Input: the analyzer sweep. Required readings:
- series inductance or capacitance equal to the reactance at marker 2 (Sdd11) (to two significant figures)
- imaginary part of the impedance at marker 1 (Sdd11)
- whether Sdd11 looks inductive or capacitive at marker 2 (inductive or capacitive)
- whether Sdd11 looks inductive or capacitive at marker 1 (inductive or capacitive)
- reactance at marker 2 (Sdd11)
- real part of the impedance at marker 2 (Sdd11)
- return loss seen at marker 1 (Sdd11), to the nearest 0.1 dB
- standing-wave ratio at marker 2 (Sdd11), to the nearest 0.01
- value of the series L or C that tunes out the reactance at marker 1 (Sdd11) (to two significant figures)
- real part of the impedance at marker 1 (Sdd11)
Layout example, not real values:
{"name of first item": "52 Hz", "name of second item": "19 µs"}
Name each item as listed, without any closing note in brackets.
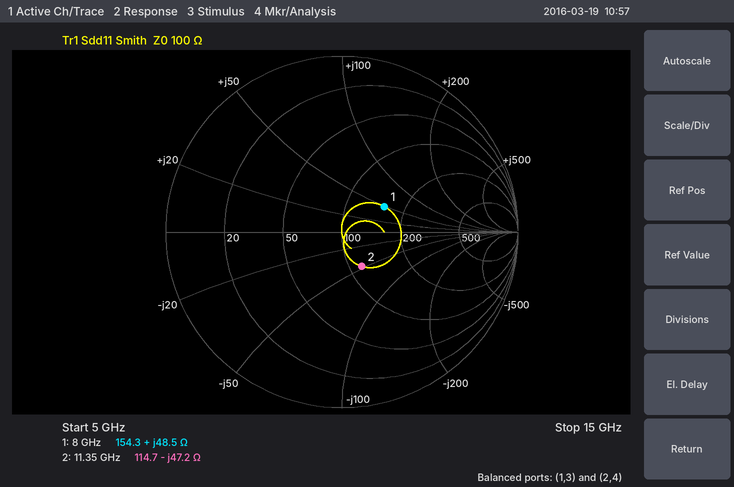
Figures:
{"series inductance or capacitance equal to the reactance at marker 2 (Sdd11)": "300 fF", "imaginary part of the impedance at marker 1": "+48.5 Ω", "whether Sdd11 looks inductive or capacitive at marker 2": "capacitive", "whether Sdd11 looks inductive or capacitive at marker 1": "inductive", "reactance at marker 2": "-47.2 Ω", "real part of the impedance at marker 2": "114.7 Ω", "return loss seen at marker 1 (Sdd11), to the nearest 0.1 dB": "11.0 dB", "standing-wave ratio at marker 2 (Sdd11), to the nearest 0.01": "1.58", "value of the series L or C that tunes out the reactance at marker 1 (Sdd11)": "410 fF", "real part of the impedance at marker 1": "154.3 Ω"}
